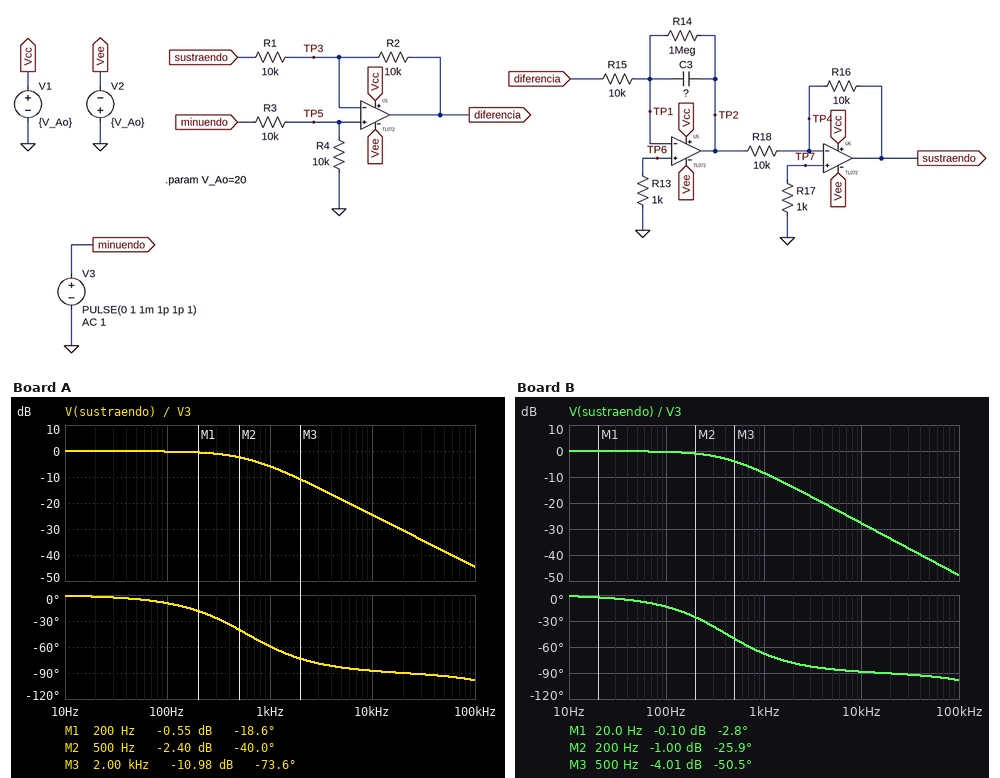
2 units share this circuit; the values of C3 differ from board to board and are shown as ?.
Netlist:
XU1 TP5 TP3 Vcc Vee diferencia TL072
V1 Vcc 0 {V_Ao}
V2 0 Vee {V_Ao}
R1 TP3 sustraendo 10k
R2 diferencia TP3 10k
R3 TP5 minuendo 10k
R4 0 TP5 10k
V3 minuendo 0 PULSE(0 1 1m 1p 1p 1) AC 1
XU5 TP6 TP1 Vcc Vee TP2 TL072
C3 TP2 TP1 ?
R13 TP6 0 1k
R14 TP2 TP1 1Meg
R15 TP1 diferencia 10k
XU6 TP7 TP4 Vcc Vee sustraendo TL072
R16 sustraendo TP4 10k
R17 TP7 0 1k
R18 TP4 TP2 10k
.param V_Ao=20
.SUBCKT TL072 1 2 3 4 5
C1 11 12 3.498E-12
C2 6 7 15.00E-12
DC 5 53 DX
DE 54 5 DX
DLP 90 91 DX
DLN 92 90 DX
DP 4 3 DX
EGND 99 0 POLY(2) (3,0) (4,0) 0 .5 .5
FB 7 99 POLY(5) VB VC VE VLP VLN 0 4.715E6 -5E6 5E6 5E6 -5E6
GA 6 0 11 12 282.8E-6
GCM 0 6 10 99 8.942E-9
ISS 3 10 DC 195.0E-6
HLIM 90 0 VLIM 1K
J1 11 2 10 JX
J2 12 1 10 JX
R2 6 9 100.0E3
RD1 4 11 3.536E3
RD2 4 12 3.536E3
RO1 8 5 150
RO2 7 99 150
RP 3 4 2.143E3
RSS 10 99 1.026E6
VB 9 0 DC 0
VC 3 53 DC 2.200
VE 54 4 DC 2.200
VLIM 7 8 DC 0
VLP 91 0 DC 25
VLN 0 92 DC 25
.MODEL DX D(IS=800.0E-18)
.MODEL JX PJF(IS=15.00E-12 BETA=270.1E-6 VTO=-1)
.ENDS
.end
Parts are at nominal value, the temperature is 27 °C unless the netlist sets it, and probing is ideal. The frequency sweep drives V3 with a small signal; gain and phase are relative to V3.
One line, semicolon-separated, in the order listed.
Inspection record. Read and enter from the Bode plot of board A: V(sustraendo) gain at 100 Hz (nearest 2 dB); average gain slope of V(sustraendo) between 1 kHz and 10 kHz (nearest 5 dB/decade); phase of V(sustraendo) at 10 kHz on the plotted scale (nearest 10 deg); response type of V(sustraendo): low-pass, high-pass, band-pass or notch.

0 dB; -20 dB/decade; -90 deg; low-pass
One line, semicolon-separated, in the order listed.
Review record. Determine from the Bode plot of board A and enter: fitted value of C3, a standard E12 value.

27 nF
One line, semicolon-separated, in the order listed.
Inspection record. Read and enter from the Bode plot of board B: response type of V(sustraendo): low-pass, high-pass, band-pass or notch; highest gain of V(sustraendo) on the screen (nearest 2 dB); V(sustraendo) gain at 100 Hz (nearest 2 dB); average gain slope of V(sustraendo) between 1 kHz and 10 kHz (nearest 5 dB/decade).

low-pass; 0 dB; 0 dB; -20 dB/decade
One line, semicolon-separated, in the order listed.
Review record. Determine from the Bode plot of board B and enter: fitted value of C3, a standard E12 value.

39 nF
